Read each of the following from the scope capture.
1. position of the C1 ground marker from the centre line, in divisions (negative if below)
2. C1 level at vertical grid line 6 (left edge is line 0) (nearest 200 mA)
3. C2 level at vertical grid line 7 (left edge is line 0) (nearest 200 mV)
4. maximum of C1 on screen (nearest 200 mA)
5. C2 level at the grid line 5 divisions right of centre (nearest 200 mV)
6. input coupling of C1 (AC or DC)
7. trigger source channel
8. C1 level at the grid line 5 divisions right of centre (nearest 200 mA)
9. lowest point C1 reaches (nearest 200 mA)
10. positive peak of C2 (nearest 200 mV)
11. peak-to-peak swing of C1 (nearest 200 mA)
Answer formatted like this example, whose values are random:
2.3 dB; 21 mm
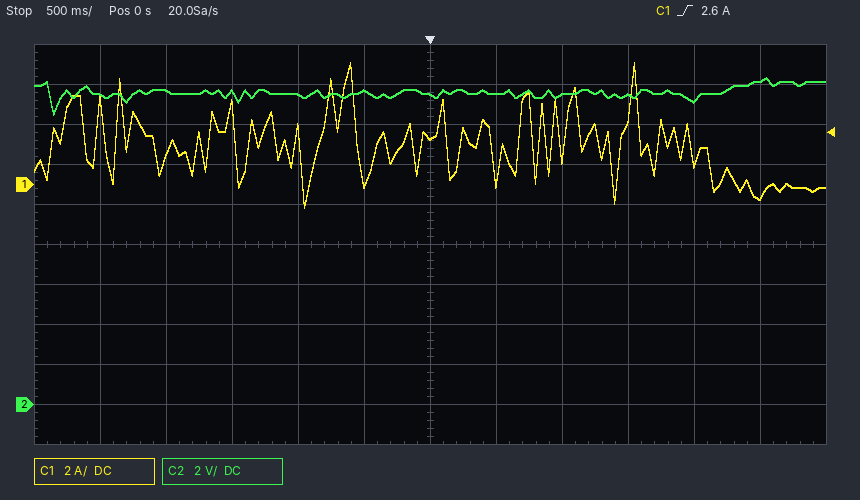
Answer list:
+1.5 div; 2.4 A; 15.6 V; 6.0 A; 16.2 V; DC; C1; -600 mA; -1.2 A; 16.4 V; 7.2 A
